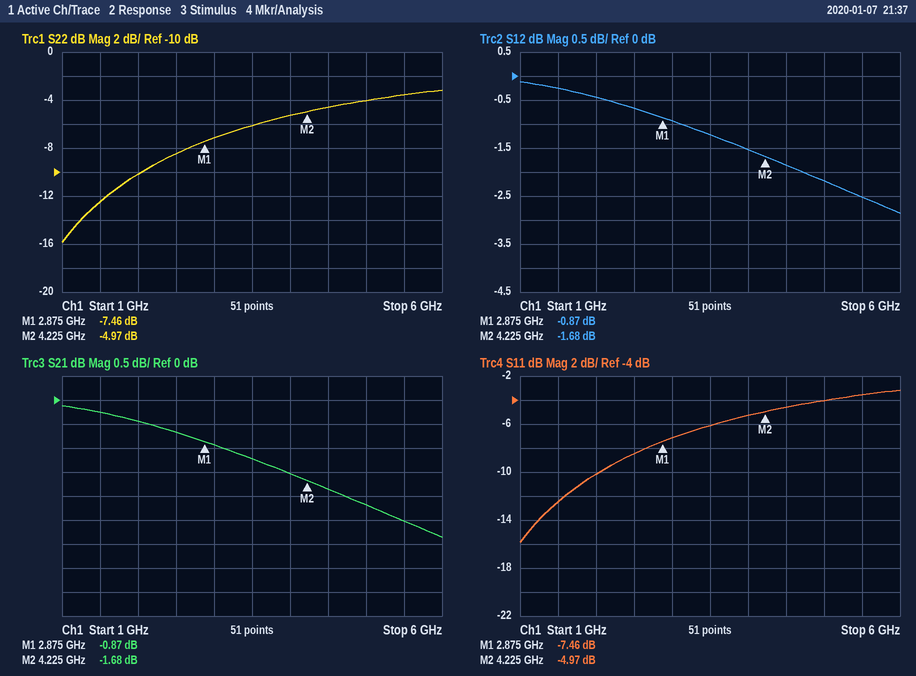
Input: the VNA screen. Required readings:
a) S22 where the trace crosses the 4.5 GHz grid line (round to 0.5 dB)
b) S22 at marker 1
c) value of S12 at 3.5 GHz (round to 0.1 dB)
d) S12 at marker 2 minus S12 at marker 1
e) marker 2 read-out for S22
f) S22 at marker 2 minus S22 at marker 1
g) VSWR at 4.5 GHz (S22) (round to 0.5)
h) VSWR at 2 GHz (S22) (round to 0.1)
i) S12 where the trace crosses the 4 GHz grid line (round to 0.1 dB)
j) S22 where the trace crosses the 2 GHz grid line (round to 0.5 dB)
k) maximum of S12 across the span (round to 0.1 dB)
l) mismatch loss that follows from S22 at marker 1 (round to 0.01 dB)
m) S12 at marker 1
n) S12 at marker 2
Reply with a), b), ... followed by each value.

a) -4.5 dB
b) -7.46 dB
c) -1.2 dB
d) -0.81 dB
e) -4.97 dB
f) 2.49 dB
g) 4.0
h) 1.9
i) -1.5 dB
j) -10.0 dB
k) -0.1 dB
l) 0.86 dB
m) -0.87 dB
n) -1.68 dB
